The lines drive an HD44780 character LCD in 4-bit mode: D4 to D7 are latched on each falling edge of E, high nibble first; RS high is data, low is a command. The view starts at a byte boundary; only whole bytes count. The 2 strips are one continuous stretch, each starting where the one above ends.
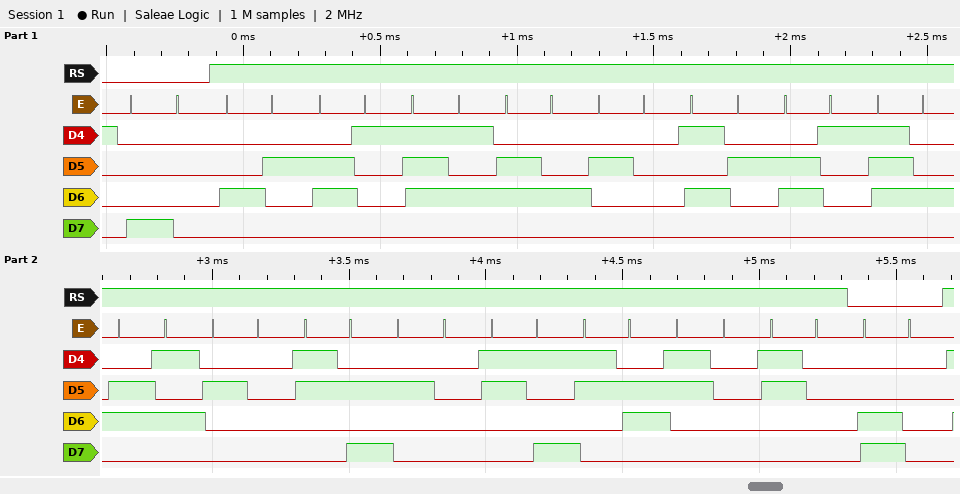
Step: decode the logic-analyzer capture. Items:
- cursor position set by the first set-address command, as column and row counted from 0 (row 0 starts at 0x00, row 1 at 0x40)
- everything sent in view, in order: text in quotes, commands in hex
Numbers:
column 0, row 0
0x80 "Baud Rate : 9600" 0xC0
